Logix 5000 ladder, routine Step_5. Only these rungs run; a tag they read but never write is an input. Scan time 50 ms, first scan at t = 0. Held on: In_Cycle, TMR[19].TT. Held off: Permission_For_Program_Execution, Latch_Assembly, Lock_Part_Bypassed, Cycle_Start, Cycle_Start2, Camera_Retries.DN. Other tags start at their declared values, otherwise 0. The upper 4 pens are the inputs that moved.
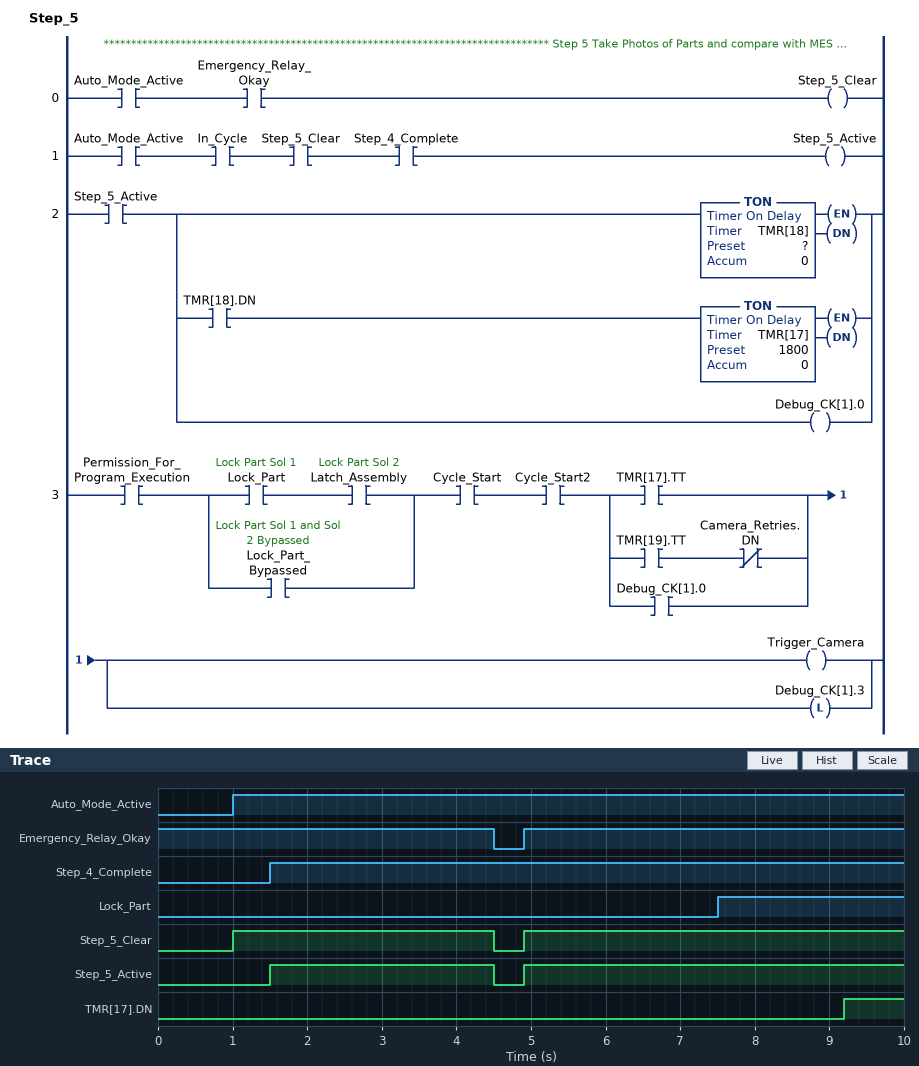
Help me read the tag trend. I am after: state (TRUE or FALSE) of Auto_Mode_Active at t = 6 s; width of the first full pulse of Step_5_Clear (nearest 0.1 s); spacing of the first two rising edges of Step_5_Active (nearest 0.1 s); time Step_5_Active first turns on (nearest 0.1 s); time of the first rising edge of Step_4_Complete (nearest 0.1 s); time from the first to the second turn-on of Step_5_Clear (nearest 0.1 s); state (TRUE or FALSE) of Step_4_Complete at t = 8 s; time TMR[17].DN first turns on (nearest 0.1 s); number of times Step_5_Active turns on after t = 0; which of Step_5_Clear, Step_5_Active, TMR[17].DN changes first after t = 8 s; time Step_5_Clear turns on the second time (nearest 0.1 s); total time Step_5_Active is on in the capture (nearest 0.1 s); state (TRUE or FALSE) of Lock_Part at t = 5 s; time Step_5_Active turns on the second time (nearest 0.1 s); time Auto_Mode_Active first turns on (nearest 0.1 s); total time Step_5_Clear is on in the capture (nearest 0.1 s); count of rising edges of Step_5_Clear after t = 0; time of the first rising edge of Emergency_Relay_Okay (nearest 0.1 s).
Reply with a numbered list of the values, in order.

1. TRUE
2. 3.5 s
3. 3.4 s
4. 1.5 s
5. 1.5 s
6. 3.9 s
7. TRUE
8. 9.2 s
9. 2
10. TMR[17].DN
11. 4.9 s
12. 8.1 s
13. FALSE
14. 4.9 s
15. 1.0 s
16. 8.6 s
17. 2
18. 4.9 s
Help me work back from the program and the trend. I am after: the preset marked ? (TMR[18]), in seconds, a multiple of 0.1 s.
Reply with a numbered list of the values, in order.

1. 2.5 s
